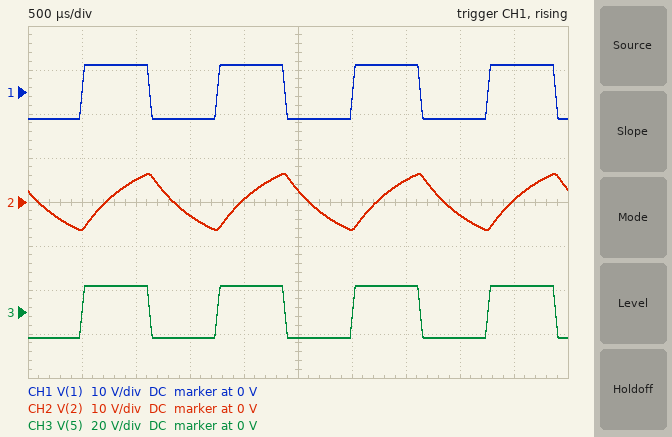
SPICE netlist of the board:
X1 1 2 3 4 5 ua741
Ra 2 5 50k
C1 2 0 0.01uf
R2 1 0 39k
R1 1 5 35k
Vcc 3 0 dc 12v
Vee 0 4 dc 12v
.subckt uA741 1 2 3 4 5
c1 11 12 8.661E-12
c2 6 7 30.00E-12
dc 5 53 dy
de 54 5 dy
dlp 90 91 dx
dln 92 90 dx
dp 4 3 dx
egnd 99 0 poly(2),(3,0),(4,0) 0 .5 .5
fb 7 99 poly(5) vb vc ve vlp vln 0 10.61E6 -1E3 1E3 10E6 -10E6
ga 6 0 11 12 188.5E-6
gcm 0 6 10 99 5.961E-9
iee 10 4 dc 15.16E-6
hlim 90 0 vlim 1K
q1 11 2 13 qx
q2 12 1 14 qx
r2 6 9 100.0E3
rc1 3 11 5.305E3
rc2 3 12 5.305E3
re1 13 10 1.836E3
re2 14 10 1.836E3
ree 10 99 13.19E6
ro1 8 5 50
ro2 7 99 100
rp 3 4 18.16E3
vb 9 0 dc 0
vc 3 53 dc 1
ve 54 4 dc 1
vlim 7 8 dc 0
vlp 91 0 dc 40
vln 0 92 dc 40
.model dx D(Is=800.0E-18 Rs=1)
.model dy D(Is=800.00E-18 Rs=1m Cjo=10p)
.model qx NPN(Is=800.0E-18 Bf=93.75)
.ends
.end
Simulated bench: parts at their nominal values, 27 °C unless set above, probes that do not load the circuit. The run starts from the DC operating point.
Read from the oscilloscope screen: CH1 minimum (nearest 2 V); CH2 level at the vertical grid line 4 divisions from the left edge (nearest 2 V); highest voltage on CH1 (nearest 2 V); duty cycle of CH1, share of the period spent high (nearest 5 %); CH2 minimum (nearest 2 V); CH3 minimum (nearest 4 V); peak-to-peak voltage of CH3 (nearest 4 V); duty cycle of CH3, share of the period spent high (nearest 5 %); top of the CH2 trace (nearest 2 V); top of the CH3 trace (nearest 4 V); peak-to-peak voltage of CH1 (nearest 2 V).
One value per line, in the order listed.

-6 V
0 V
6 V
50 %
-6 V
-12 V
24 V
50 %
6 V
12 V
12 V
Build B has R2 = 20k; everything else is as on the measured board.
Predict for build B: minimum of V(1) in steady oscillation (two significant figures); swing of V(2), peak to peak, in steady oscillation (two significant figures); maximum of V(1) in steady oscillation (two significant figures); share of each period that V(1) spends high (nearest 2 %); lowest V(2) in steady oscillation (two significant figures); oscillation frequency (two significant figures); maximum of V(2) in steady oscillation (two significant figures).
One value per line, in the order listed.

-4.3 V
9.0 V
4.3 V
50 %
-4.5 V
1.2 kHz
4.5 V
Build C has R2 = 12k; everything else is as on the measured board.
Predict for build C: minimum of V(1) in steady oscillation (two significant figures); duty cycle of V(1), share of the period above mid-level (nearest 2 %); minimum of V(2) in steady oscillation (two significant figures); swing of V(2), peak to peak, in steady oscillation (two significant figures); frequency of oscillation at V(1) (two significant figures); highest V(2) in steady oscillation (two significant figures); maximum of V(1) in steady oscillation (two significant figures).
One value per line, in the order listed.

-3.0 V
50 %
-3.3 V
6.6 V
1.6 kHz
3.3 V
3.0 V
